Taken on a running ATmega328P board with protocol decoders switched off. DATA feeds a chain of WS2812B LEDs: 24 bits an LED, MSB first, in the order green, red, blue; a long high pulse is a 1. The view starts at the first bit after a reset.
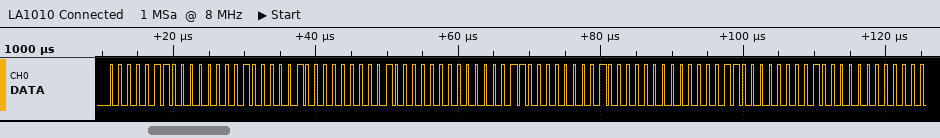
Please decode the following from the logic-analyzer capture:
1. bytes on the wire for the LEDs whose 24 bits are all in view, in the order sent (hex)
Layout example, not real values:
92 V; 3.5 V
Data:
06 01 04 01 00 06 01 00 06
